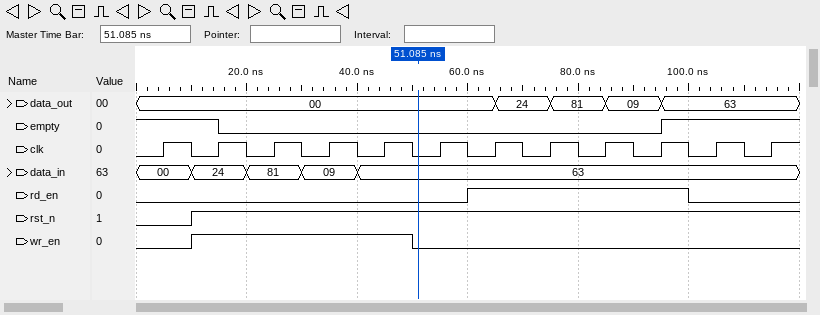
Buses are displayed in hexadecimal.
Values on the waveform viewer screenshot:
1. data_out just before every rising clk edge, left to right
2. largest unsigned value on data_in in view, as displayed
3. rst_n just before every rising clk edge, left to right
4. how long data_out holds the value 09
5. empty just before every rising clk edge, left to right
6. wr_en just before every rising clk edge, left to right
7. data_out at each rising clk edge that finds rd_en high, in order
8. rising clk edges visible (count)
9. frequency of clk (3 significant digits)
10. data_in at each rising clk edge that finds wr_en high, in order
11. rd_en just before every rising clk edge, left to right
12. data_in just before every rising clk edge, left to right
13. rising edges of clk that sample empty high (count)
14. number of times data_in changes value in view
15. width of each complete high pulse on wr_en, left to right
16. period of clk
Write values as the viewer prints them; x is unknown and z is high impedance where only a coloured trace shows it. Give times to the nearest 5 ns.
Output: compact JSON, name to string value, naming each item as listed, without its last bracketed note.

{"data_out just before every rising clk edge, left to right": "00, 00, 00, 00, 00, 00, 00, 24, 81, 09, 63, 63", "largest unsigned value on data_in in view, as displayed": "81", "rst_n just before every rising clk edge, left to right": "0 1 1 1 1 1 1 1 1 1 1 1", "how long data_out holds the value 09": "10 ns", "empty just before every rising clk edge, left to right": "1 1 0 0 0 0 0 0 0 0 1 1", "wr_en just before every rising clk edge, left to right": "0 1 1 1 1 0 0 0 0 0 0 0", "data_out at each rising clk edge that finds rd_en high, in order": "00, 24, 81, 09", "rising clk edges visible": "12", "frequency of clk": "100 MHz", "data_in at each rising clk edge that finds wr_en high, in order": "24, 81, 09, 63", "rd_en just before every rising clk edge, left to right": "0 0 0 0 0 0 1 1 1 1 0 0", "data_in just before every rising clk edge, left to right": "00, 24, 81, 09, 63, 63, 63, 63, 63, 63, 63, 63", "rising edges of clk that sample empty high": "4", "number of times data_in changes value in view": "4", "width of each complete high pulse on wr_en, left to right": "40 ns", "period of clk": "10 ns"}
